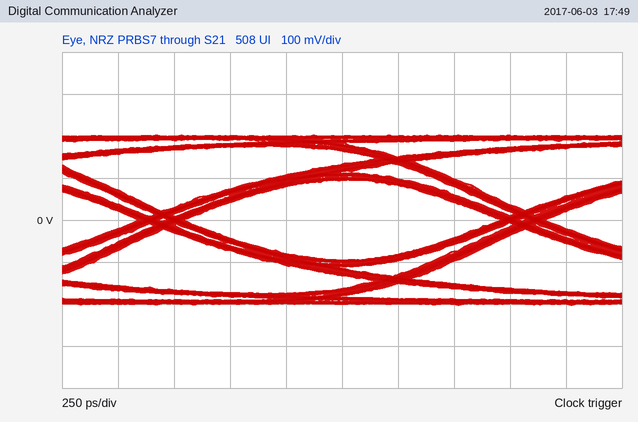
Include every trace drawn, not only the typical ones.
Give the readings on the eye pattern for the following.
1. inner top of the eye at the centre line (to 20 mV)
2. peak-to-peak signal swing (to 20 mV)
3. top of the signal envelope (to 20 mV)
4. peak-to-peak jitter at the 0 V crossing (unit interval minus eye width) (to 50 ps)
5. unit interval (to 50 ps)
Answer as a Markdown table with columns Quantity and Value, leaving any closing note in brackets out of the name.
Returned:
| Quantity | Value |
|---|---|
| inner top of the eye at the centre line | 100 mV |
| peak-to-peak signal swing | 400 mV |
| top of the signal envelope | 200 mV |
| peak-to-peak jitter at the 0 V crossing (unit interval minus eye width) | 200 ps |
| unit interval | 1.60 ns |
